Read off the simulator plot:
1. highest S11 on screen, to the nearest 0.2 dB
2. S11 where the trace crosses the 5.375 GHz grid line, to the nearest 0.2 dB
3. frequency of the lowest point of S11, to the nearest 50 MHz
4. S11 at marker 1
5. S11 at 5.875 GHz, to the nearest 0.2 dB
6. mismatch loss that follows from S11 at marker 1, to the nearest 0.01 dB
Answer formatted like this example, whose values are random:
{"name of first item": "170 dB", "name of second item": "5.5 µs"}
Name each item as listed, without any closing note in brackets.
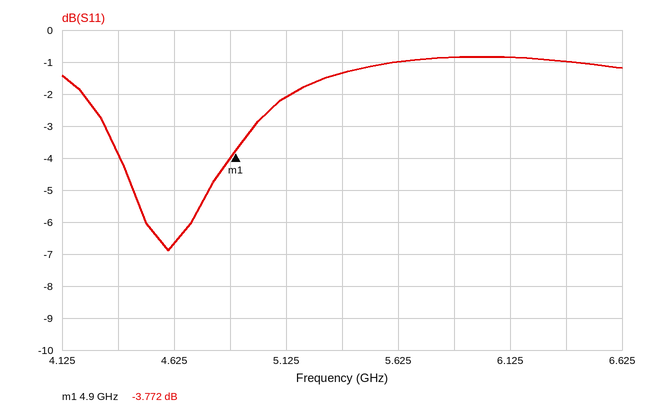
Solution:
{"highest S11 on screen, to the nearest 0.2 dB": "-0.8 dB", "S11 where the trace crosses the 5.375 GHz grid line, to the nearest 0.2 dB": "-1.4 dB", "frequency of the lowest point of S11, to the nearest 50 MHz": "4.60 GHz", "S11 at marker 1": "-3.772 dB", "S11 at 5.875 GHz, to the nearest 0.2 dB": "-0.8 dB", "mismatch loss that follows from S11 at marker 1, to the nearest 0.01 dB": "2.36 dB"}
